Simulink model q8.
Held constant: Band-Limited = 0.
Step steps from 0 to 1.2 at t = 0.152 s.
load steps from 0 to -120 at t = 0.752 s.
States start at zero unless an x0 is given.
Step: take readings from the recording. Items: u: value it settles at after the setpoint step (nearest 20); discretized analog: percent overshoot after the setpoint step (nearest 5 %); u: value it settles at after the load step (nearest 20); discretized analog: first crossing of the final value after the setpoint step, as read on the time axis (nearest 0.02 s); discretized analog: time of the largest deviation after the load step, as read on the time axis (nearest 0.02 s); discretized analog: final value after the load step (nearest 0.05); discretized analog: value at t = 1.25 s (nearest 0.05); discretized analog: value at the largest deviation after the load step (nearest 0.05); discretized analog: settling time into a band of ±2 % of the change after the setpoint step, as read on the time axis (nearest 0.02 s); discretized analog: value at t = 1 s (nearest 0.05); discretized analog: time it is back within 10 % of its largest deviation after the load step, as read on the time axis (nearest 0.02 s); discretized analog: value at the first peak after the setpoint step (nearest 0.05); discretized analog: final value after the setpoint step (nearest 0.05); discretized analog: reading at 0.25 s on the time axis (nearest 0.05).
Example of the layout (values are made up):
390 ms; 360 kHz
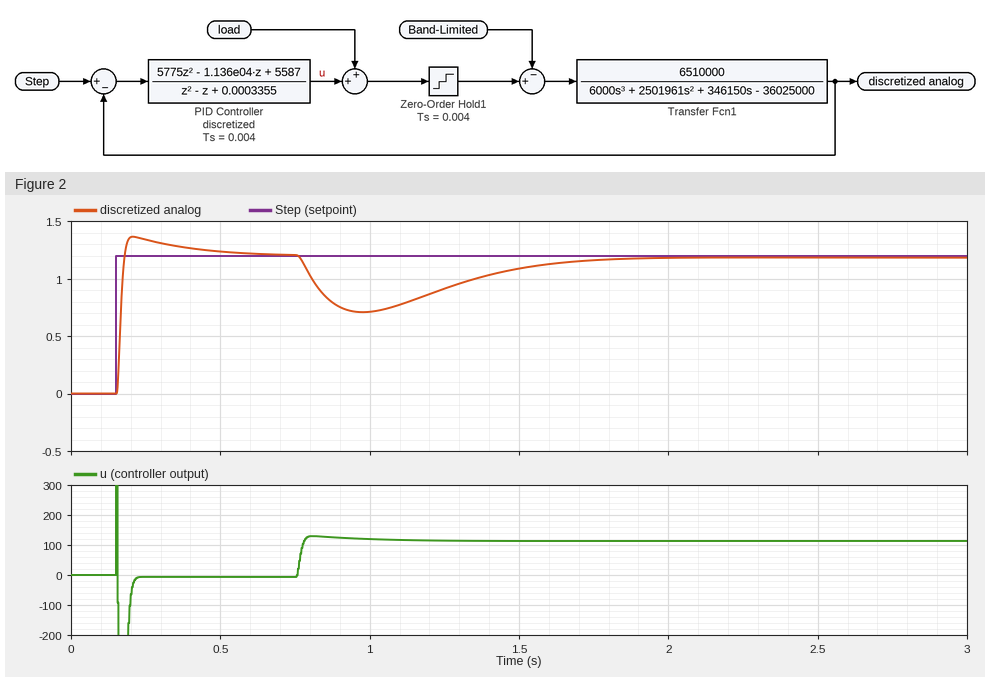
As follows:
0; 15 %; 120; 0.18 s; 0.98 s; 1.20; 0.90; 0.70; 0.54 s; 0.70; 1.62 s; 1.35; 1.20; 1.35
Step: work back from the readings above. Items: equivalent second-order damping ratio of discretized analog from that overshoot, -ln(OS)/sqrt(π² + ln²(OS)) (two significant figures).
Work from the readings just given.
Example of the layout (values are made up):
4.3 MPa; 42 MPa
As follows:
0.52
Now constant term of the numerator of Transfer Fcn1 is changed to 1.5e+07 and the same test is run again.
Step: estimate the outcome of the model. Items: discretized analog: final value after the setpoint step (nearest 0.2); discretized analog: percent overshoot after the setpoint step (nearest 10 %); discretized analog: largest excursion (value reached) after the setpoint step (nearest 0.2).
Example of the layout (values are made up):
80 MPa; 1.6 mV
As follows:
1.2; 40 %; 1.6
